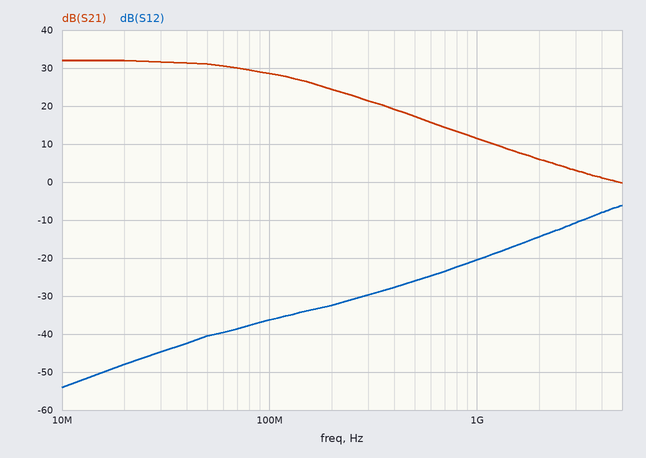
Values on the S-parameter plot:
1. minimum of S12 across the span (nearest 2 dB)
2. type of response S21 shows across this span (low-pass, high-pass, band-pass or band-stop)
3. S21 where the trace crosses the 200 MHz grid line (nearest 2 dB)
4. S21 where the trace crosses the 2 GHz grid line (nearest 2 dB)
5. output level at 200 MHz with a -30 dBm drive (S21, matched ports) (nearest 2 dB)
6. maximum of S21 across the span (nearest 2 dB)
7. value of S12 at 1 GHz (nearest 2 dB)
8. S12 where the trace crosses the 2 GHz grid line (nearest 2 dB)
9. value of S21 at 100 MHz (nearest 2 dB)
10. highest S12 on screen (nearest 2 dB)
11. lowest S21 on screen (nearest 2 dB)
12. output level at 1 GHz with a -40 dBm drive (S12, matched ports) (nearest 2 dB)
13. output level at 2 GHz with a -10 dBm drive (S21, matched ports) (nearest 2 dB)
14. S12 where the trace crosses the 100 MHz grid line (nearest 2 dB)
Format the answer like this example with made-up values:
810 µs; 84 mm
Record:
-54 dB; low-pass; 24 dB; 6 dB; -6 dBm; 32 dB; -20 dB; -14 dB; 28 dB; -6 dB; 0 dB; -60 dBm; -4 dBm; -36 dB
